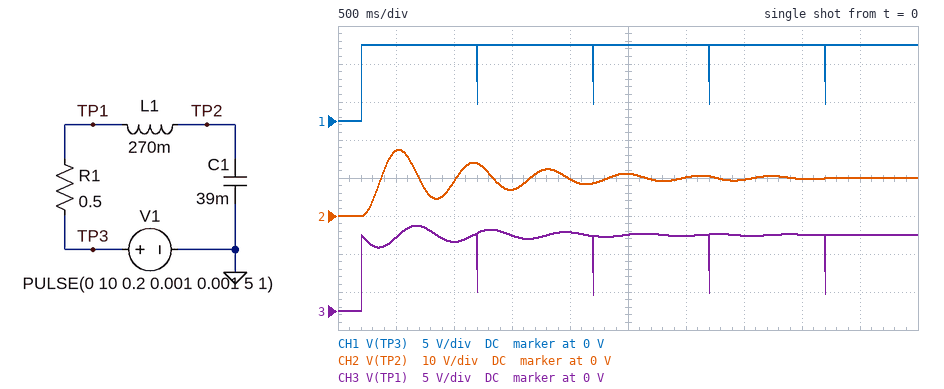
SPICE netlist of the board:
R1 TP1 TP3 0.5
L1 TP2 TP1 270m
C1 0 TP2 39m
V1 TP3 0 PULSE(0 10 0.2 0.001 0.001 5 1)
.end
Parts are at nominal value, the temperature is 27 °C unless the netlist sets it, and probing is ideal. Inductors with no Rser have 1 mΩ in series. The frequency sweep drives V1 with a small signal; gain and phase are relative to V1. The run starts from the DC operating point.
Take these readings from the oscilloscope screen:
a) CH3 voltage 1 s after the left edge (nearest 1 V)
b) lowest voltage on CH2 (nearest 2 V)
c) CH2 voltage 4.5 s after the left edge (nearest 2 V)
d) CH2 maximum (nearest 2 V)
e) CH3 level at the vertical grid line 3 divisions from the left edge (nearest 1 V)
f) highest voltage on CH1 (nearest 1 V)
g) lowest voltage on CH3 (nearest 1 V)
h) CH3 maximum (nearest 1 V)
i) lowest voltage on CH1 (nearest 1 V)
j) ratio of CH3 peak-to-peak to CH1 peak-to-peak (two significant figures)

9 V
0 V
10 V
18 V
10 V
10 V
0 V
11 V
0 V
1.1
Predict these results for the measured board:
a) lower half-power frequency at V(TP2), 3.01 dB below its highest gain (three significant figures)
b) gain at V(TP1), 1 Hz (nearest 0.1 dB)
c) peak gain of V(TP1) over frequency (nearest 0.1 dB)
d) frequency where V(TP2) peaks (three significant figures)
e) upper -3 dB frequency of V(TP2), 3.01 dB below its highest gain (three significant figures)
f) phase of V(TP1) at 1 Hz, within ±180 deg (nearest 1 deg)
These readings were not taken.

1.38 Hz
-0.2 dB
0 dB
1.54 Hz
1.68 Hz
-12 deg
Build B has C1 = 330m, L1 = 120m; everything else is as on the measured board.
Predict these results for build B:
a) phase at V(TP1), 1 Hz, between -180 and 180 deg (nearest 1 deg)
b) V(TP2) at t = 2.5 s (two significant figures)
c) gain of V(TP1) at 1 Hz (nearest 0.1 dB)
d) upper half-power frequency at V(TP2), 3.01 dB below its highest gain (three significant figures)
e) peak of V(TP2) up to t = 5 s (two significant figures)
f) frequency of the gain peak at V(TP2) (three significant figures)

61 deg
10 V
-6.4 dB
950 mHz
12 V
647 mHz
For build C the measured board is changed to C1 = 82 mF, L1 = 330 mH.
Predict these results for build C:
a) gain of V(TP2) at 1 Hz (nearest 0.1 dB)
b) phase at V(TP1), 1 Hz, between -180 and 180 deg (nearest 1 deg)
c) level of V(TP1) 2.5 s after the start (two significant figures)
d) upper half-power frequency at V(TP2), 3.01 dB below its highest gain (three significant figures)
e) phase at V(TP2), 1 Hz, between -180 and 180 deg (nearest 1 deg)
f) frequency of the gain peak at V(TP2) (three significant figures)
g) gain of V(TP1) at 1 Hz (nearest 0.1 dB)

11.5 dB
75 deg
9.6 V
1.07 Hz
-105 deg
952 mHz
-11.8 dB
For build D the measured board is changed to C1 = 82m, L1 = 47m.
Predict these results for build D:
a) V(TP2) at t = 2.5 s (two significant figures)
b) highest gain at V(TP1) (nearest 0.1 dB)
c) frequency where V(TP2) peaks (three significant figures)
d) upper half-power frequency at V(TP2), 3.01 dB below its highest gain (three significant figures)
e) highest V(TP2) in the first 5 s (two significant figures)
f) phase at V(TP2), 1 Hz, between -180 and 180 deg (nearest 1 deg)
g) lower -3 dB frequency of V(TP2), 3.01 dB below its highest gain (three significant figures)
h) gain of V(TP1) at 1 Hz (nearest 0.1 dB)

10 V
0 dB
2.27 Hz
3.04 Hz
13 V
-17 deg
1.01 Hz
-0.4 dB
